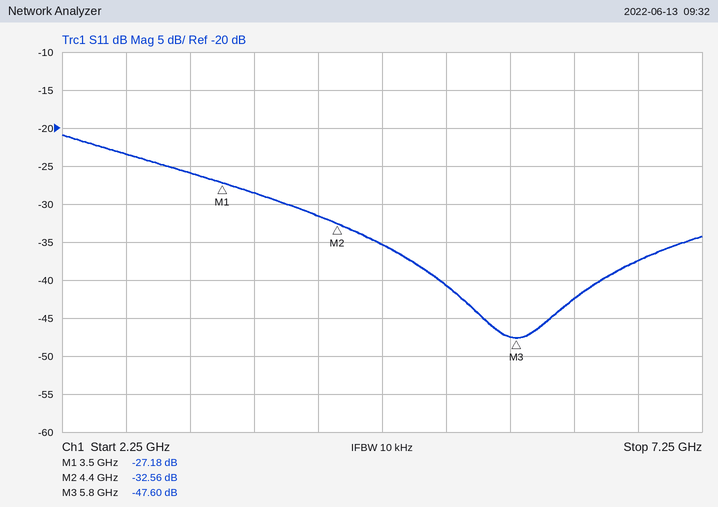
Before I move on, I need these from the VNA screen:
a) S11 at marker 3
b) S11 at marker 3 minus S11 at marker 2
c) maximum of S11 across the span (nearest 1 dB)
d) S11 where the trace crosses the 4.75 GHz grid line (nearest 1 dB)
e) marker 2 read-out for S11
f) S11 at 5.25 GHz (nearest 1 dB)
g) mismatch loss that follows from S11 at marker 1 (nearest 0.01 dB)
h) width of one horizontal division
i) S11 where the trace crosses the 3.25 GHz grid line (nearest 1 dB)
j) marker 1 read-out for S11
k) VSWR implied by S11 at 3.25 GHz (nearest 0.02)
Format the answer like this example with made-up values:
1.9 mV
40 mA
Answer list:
-47.60 dB
-15.04 dB
-21 dB
-35 dB
-32.56 dB
-41 dB
0.01 dB
500 MHz
-26 dB
-27.18 dB
1.10
